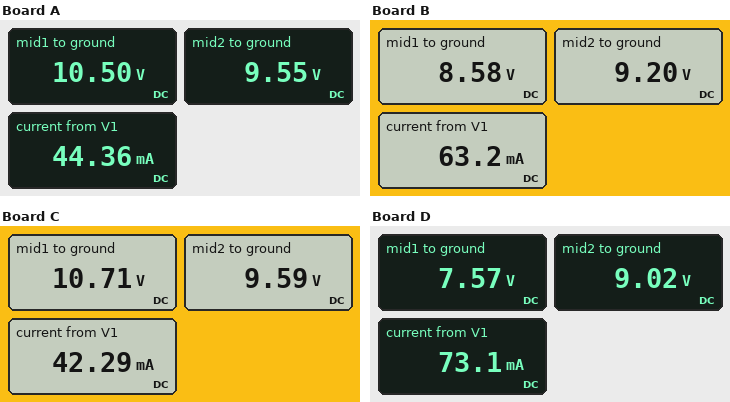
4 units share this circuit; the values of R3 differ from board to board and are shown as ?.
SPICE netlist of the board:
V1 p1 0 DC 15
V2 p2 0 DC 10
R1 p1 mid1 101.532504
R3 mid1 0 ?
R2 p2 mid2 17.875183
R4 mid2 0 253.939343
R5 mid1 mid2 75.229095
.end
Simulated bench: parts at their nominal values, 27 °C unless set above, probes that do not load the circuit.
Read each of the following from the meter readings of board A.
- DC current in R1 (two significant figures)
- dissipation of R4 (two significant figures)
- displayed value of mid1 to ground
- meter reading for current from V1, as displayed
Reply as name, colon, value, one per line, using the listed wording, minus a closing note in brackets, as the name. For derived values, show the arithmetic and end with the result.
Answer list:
DC current in R1: (15 V - 10.5 V) / 101.5 Ω = 44 mA
dissipation of R4: (9.55 V)^2 / 253.9 Ω = 360 mW
displayed value of mid1 to ground: 10.50 V
meter reading for current from V1, as displayed: 44.36 mA
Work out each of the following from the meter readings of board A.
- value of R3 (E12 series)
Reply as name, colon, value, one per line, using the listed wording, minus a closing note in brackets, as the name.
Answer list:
value of R3: 330 Ω
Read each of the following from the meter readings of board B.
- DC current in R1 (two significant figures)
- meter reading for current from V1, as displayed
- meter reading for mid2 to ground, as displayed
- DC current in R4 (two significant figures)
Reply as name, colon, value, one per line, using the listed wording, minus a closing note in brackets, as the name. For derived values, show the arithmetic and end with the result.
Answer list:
DC current in R1: (15 V - 8.58 V) / 101.5 Ω = 63 mA
meter reading for current from V1, as displayed: 63.2 mA
meter reading for mid2 to ground, as displayed: 9.20 V
DC current in R4: (9.2 V) / 253.9 Ω = 36 mA
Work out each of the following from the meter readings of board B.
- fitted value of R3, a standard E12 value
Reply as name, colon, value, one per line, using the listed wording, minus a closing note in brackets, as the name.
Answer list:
fitted value of R3, a standard E12 value: 120 Ω
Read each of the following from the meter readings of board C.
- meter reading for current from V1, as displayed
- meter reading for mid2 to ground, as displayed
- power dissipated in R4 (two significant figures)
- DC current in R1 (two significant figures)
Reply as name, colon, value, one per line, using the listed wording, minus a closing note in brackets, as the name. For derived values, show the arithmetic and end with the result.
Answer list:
meter reading for current from V1, as displayed: 42.29 mA
meter reading for mid2 to ground, as displayed: 9.59 V
power dissipated in R4: (9.59 V)^2 / 253.9 Ω = 360 mW
DC current in R1: (15 V - 10.71 V) / 101.5 Ω = 42 mA
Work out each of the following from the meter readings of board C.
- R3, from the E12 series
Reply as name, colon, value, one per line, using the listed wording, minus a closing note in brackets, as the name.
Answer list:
R3, from the E12 series: 390 Ω
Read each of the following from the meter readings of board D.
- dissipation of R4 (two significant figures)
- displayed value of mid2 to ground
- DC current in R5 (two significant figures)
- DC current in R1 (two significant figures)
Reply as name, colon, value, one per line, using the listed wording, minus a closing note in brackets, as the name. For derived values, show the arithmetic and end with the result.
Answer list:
dissipation of R4: (9.02 V)^2 / 253.9 Ω = 320 mW
displayed value of mid2 to ground: 9.02 V
DC current in R5: (9.02 V - 7.57 V) / 75.23 Ω = 19 mA
DC current in R1: (15 V - 7.57 V) / 101.5 Ω = 73 mA
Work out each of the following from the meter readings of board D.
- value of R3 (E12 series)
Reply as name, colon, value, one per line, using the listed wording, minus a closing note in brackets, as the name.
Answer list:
value of R3: 82 Ω
